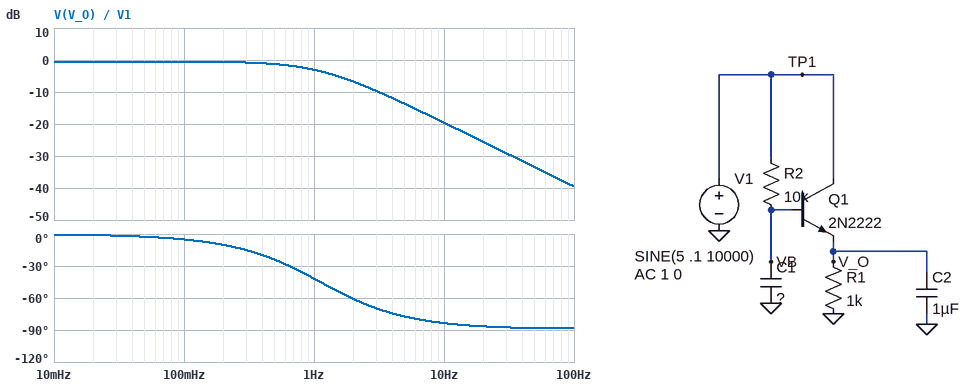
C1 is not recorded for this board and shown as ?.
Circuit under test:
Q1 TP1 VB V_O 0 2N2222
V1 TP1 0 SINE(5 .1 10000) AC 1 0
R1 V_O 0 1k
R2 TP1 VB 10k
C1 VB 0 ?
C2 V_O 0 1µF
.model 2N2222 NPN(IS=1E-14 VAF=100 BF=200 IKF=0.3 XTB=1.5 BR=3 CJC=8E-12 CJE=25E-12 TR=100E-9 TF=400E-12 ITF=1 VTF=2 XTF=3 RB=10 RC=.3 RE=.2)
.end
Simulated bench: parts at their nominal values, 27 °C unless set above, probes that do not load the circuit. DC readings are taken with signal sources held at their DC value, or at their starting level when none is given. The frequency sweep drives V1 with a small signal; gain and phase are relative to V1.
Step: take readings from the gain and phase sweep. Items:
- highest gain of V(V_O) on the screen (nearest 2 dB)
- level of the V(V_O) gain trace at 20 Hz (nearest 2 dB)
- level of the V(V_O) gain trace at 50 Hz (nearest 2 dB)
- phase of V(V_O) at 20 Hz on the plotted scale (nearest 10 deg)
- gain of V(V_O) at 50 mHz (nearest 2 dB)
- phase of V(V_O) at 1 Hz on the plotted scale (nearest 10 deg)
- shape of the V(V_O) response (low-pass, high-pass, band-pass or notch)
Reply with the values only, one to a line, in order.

0 dB
-26 dB
-34 dB
-90 deg
0 dB
-40 deg
low-pass
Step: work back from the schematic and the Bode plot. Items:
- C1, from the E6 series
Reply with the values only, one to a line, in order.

15 µF
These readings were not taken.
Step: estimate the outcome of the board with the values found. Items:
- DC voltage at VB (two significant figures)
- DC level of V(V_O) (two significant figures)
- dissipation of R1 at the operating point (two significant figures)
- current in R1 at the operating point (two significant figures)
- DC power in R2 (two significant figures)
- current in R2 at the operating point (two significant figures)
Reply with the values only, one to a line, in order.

4.8 V
4.1 V
17 mW
4.1 mA
4.3 µW
21 µA
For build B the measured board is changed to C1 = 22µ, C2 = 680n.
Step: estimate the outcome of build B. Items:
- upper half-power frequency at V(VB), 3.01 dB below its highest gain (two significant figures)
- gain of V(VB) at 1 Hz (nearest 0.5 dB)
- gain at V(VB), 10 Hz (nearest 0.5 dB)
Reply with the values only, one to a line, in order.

760 mHz
-5.0 dB
-23.0 dB
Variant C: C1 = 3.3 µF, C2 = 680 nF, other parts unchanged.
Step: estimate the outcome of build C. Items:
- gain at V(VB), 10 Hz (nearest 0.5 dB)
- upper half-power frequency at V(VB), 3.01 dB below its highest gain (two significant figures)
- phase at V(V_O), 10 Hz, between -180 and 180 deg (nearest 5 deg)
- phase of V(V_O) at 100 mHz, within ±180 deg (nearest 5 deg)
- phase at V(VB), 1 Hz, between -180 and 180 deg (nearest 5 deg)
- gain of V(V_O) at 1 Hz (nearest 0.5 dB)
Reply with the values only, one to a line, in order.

-7.5 dB
5.1 Hz
-65 deg
0 deg
-10 deg
-0.5 dB
